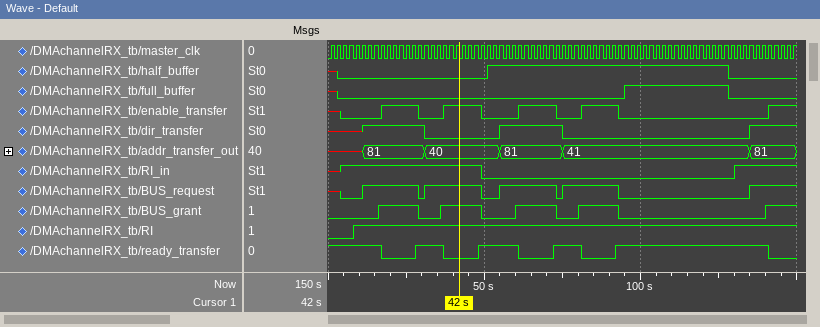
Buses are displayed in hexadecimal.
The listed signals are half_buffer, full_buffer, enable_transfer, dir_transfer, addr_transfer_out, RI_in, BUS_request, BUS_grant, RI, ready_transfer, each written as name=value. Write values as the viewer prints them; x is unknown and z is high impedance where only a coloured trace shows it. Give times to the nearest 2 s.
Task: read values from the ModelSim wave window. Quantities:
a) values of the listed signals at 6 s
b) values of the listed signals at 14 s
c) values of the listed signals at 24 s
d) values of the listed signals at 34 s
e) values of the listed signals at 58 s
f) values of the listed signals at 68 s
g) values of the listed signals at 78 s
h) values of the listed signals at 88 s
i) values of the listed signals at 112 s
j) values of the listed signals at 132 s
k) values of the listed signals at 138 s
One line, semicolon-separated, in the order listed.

half_buffer=0, full_buffer=0, enable_transfer=0, dir_transfer=x, addr_transfer_out=x, RI_in=1, BUS_request=0, BUS_grant=0, RI=0, ready_transfer=1; half_buffer=0, full_buffer=0, enable_transfer=0, dir_transfer=1, addr_transfer_out=81, RI_in=1, BUS_request=1, BUS_grant=0, RI=1, ready_transfer=1; half_buffer=0, full_buffer=0, enable_transfer=1, dir_transfer=1, addr_transfer_out=81, RI_in=1, BUS_request=1, BUS_grant=1, RI=1, ready_transfer=0; half_buffer=0, full_buffer=0, enable_transfer=0, dir_transfer=0, addr_transfer_out=40, RI_in=1, BUS_request=1, BUS_grant=0, RI=1, ready_transfer=1; half_buffer=1, full_buffer=0, enable_transfer=0, dir_transfer=1, addr_transfer_out=81, RI_in=0, BUS_request=1, BUS_grant=0, RI=1, ready_transfer=1; half_buffer=1, full_buffer=0, enable_transfer=1, dir_transfer=1, addr_transfer_out=81, RI_in=0, BUS_request=1, BUS_grant=1, RI=1, ready_transfer=0; half_buffer=1, full_buffer=0, enable_transfer=0, dir_transfer=0, addr_transfer_out=41, RI_in=0, BUS_request=1, BUS_grant=0, RI=1, ready_transfer=1; half_buffer=1, full_buffer=0, enable_transfer=1, dir_transfer=0, addr_transfer_out=41, RI_in=0, BUS_request=1, BUS_grant=1, RI=1, ready_transfer=0; half_buffer=1, full_buffer=1, enable_transfer=0, dir_transfer=0, addr_transfer_out=41, RI_in=0, BUS_request=0, BUS_grant=0, RI=1, ready_transfer=1; half_buffer=0, full_buffer=0, enable_transfer=0, dir_transfer=0, addr_transfer_out=41, RI_in=1, BUS_request=0, BUS_grant=0, RI=1, ready_transfer=1; half_buffer=0, full_buffer=0, enable_transfer=0, dir_transfer=1, addr_transfer_out=81, RI_in=1, BUS_request=1, BUS_grant=0, RI=1, ready_transfer=1
